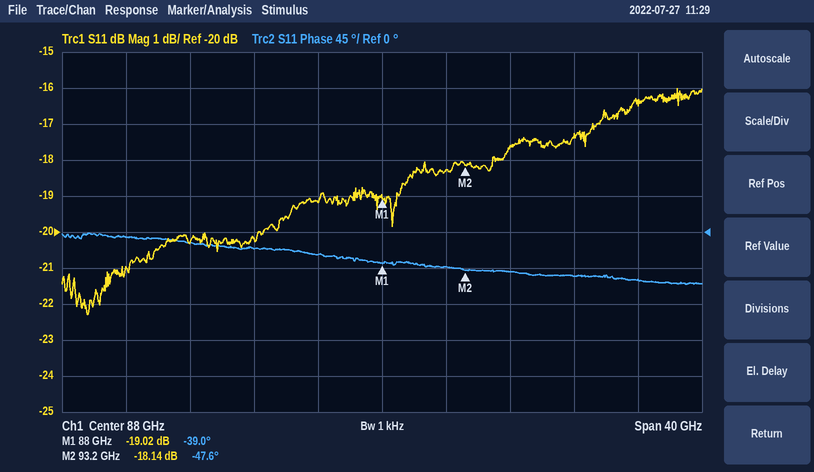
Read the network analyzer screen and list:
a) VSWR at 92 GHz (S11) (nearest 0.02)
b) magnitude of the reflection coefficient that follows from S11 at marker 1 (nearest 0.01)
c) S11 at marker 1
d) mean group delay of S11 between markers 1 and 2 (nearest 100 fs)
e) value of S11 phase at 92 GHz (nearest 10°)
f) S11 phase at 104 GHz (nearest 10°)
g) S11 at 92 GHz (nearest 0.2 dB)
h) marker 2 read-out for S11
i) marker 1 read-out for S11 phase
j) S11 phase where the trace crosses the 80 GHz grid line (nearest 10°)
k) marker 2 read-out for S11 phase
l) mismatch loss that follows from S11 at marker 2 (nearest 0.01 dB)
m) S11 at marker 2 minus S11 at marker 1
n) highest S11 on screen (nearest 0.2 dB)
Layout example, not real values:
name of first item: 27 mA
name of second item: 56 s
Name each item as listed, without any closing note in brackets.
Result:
VSWR at 92 GHz (S11): 1.28
magnitude of the reflection coefficient that follows from S11 at marker 1: 0.11
S11 at marker 1: -19.02 dB
mean group delay of S11 between markers 1 and 2: 4.6 ps
value of S11 phase at 92 GHz: -40°
S11 phase at 104 GHz: -60°
S11 at 92 GHz: -18.2 dB
marker 2 read-out for S11: -18.14 dB
marker 1 read-out for S11 phase: -39.0°
S11 phase where the trace crosses the 80 GHz grid line: -20°
marker 2 read-out for S11 phase: -47.6°
mismatch loss that follows from S11 at marker 2: 0.07 dB
S11 at marker 2 minus S11 at marker 1: 0.88 dB
highest S11 on screen: -16.0 dB
